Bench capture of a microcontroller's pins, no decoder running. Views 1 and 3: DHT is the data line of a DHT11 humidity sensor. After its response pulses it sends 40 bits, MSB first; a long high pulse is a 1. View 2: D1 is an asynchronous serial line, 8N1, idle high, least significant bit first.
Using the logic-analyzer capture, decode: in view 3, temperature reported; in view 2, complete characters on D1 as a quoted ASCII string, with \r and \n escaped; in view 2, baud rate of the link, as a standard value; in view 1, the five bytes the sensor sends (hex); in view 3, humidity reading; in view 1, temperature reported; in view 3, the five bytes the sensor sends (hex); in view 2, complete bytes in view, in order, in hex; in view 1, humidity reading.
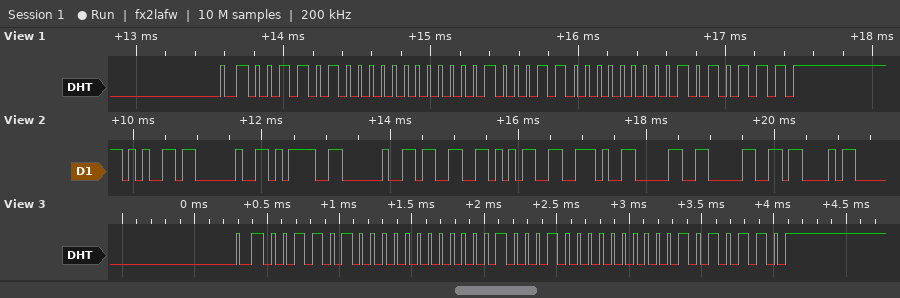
34.0 °C
"e = 35.00C"
9600 baud
34 00 23 00 57
52 %
35.0 °C
34 00 22 00 56
65 20 3D 20 33 35 2E 30 30 43
52 %
